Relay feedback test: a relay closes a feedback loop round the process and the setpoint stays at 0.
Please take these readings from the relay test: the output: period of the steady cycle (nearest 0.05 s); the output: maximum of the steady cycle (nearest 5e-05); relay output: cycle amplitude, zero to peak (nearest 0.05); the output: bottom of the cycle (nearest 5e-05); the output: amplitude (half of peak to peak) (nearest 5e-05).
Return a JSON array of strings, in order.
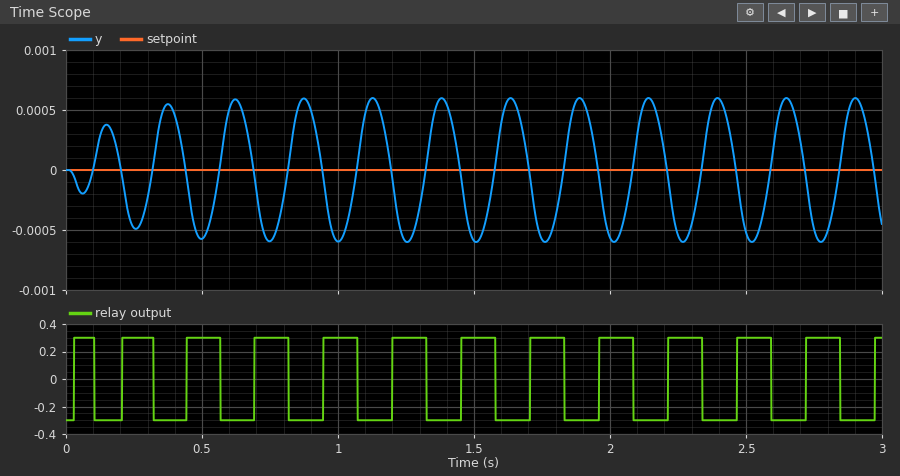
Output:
["0.25 s", "0.00060", "0.30", "-0.00060", "0.00060"]
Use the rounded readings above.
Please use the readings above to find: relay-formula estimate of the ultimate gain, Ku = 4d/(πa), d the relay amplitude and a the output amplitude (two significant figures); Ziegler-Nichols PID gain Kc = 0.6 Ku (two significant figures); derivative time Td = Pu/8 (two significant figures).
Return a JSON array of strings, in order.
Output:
["640", "380", "0.031 s"]
